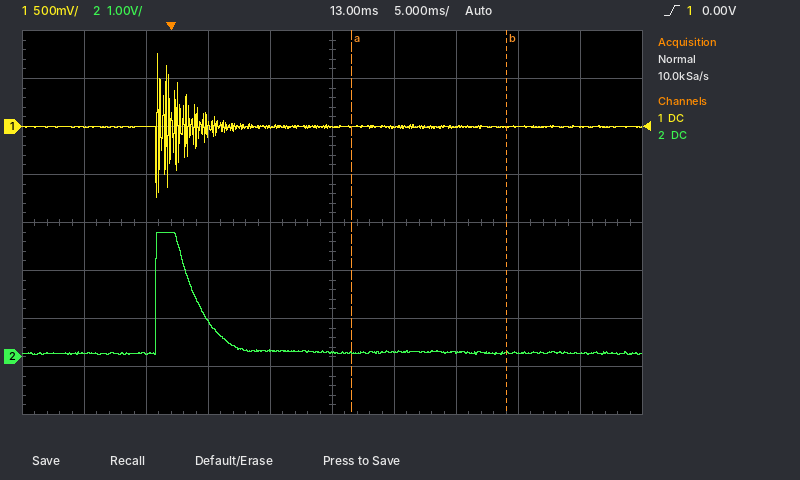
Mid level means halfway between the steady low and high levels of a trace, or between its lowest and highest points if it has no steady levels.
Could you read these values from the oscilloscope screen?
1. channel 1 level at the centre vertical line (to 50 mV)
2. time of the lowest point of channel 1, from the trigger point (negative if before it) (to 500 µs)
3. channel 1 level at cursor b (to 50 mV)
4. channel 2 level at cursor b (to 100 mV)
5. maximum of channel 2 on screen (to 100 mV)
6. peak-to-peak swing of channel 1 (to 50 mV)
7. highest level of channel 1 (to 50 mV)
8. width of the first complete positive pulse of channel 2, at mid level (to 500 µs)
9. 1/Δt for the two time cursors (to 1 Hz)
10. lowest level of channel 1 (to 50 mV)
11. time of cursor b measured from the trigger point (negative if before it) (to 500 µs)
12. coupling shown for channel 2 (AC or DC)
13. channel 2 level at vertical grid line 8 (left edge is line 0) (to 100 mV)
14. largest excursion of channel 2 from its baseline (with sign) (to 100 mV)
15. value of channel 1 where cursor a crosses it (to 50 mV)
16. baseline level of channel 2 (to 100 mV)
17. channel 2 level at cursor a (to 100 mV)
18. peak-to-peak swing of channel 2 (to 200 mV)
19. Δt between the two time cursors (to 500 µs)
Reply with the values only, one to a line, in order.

0 mV
-1.0 ms
0 mV
100 mV
2.6 V
1.50 V
750 mV
3.0 ms
80 Hz
-750 mV
+27.0 ms
DC
100 mV
+2.5 V
0 mV
100 mV
100 mV
2.6 V
12.5 ms
